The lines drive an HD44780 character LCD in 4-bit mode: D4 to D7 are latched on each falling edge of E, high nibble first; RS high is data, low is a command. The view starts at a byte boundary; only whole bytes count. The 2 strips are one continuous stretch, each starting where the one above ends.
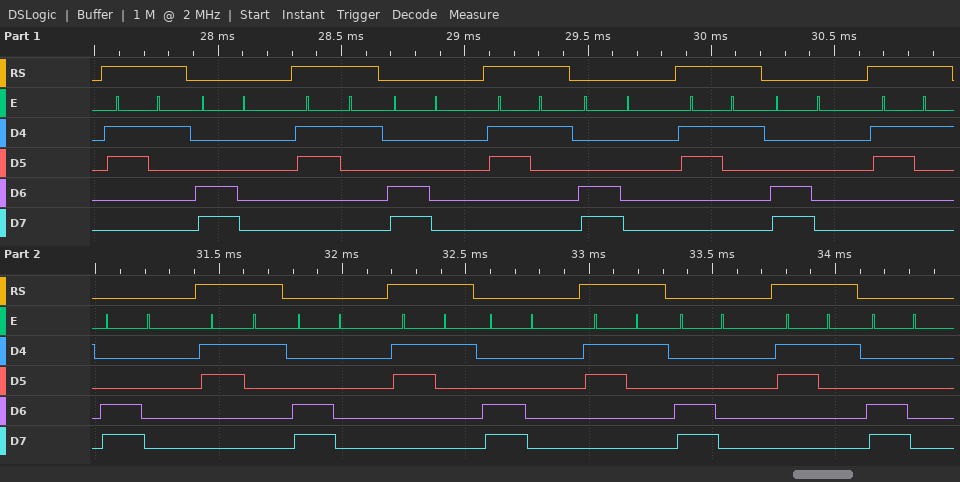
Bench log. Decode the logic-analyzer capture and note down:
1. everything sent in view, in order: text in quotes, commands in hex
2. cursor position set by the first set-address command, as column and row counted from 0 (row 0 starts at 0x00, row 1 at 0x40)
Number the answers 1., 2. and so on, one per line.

1. "1" 0xC0 "1" 0xC0 "1" 0xC0 "1" 0xC0 "1" 0xC0 "1" 0xC0 "1" 0xC0 "1" 0xC0 "1" 0xC0
2. column 0, row 1
